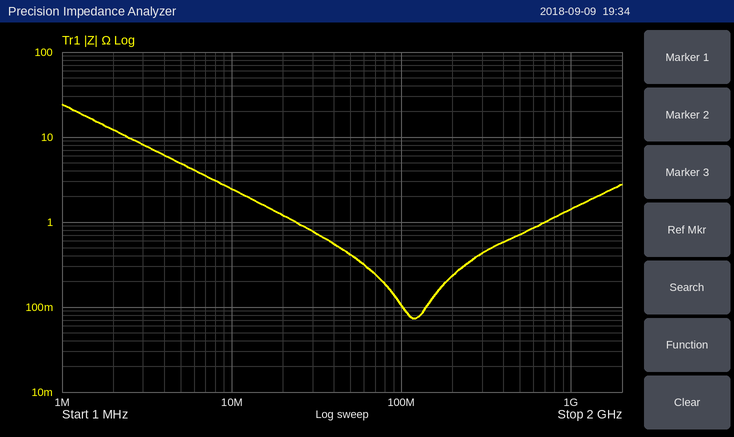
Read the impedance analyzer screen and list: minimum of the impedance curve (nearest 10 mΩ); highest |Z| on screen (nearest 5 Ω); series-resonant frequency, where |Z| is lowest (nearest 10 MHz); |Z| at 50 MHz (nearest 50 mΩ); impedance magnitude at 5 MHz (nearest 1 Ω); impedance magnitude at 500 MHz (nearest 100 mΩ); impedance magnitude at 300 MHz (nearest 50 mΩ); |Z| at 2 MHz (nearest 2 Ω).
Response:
70 mΩ
25 Ω
120 MHz
400 mΩ
5 Ω
700 mΩ
450 mΩ
12 Ω
